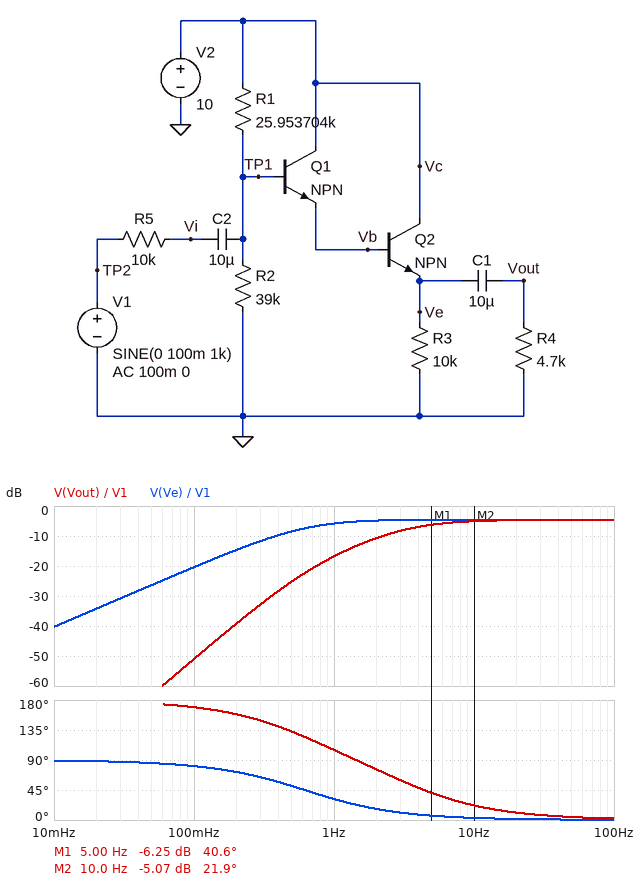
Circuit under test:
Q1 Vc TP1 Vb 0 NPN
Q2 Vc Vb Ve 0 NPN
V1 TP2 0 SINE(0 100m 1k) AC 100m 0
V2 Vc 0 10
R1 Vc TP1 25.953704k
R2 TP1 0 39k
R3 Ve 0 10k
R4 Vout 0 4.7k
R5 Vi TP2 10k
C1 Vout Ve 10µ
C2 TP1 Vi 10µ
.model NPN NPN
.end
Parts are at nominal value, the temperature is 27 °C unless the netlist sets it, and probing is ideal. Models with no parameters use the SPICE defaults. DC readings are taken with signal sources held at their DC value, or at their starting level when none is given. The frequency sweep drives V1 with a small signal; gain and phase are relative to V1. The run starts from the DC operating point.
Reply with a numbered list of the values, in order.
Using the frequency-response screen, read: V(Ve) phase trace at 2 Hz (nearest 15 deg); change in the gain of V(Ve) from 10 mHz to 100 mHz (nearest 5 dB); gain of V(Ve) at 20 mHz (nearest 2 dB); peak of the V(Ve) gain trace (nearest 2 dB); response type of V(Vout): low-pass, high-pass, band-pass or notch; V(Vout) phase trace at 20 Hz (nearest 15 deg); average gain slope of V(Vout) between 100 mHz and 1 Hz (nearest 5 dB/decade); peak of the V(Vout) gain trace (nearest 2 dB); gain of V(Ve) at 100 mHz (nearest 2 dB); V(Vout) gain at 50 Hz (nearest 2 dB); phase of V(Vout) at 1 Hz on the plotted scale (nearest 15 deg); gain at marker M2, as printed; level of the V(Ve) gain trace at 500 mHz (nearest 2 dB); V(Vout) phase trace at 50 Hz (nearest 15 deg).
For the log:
1. 15 deg
2. 20 dB
3. -34 dB
4. -4 dB
5. high-pass
6. 15 deg
7. 35 dB/decade
8. -4 dB
9. -20 dB
10. -4 dB
11. 105 deg
12. -5.07 dB
13. -8 dB
14. 0 deg
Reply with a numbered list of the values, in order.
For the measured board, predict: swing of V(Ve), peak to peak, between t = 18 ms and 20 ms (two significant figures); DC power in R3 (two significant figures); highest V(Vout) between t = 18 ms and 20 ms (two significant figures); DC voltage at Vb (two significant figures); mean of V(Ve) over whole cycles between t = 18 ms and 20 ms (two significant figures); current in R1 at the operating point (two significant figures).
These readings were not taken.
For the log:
1. 120 mV
2. 2.1 mW
3. 59 mV
4. 5.4 V
5. 4.6 V
6. 150 µA
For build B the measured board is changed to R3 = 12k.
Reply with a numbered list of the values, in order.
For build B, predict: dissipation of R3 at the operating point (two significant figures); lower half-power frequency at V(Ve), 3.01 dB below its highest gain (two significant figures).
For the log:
1. 1.8 mW
2. 590 mHz
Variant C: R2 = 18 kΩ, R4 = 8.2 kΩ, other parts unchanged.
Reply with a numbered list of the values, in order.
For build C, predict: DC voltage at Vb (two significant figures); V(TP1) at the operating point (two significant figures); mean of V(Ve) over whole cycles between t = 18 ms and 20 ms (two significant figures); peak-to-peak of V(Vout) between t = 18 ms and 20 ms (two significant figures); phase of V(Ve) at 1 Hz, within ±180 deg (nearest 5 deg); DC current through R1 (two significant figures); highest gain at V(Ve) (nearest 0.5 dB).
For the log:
1. 3.5 V
2. 4.1 V
3. 2.7 V
4. 99 mV
5. 35 deg
6. 230 µA
7. -6.0 dB
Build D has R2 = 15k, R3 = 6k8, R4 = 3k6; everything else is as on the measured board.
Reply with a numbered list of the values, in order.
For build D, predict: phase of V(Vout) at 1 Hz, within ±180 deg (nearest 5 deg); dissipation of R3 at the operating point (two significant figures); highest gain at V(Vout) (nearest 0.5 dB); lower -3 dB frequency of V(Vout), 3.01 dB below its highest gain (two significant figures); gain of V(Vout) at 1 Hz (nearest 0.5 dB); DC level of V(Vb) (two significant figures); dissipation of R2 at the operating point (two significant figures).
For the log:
1. 115 deg
2. 770 µW
3. -7.0 dB
4. 4.4 Hz
5. -22.0 dB
6. 3.0 V
7. 890 µW
